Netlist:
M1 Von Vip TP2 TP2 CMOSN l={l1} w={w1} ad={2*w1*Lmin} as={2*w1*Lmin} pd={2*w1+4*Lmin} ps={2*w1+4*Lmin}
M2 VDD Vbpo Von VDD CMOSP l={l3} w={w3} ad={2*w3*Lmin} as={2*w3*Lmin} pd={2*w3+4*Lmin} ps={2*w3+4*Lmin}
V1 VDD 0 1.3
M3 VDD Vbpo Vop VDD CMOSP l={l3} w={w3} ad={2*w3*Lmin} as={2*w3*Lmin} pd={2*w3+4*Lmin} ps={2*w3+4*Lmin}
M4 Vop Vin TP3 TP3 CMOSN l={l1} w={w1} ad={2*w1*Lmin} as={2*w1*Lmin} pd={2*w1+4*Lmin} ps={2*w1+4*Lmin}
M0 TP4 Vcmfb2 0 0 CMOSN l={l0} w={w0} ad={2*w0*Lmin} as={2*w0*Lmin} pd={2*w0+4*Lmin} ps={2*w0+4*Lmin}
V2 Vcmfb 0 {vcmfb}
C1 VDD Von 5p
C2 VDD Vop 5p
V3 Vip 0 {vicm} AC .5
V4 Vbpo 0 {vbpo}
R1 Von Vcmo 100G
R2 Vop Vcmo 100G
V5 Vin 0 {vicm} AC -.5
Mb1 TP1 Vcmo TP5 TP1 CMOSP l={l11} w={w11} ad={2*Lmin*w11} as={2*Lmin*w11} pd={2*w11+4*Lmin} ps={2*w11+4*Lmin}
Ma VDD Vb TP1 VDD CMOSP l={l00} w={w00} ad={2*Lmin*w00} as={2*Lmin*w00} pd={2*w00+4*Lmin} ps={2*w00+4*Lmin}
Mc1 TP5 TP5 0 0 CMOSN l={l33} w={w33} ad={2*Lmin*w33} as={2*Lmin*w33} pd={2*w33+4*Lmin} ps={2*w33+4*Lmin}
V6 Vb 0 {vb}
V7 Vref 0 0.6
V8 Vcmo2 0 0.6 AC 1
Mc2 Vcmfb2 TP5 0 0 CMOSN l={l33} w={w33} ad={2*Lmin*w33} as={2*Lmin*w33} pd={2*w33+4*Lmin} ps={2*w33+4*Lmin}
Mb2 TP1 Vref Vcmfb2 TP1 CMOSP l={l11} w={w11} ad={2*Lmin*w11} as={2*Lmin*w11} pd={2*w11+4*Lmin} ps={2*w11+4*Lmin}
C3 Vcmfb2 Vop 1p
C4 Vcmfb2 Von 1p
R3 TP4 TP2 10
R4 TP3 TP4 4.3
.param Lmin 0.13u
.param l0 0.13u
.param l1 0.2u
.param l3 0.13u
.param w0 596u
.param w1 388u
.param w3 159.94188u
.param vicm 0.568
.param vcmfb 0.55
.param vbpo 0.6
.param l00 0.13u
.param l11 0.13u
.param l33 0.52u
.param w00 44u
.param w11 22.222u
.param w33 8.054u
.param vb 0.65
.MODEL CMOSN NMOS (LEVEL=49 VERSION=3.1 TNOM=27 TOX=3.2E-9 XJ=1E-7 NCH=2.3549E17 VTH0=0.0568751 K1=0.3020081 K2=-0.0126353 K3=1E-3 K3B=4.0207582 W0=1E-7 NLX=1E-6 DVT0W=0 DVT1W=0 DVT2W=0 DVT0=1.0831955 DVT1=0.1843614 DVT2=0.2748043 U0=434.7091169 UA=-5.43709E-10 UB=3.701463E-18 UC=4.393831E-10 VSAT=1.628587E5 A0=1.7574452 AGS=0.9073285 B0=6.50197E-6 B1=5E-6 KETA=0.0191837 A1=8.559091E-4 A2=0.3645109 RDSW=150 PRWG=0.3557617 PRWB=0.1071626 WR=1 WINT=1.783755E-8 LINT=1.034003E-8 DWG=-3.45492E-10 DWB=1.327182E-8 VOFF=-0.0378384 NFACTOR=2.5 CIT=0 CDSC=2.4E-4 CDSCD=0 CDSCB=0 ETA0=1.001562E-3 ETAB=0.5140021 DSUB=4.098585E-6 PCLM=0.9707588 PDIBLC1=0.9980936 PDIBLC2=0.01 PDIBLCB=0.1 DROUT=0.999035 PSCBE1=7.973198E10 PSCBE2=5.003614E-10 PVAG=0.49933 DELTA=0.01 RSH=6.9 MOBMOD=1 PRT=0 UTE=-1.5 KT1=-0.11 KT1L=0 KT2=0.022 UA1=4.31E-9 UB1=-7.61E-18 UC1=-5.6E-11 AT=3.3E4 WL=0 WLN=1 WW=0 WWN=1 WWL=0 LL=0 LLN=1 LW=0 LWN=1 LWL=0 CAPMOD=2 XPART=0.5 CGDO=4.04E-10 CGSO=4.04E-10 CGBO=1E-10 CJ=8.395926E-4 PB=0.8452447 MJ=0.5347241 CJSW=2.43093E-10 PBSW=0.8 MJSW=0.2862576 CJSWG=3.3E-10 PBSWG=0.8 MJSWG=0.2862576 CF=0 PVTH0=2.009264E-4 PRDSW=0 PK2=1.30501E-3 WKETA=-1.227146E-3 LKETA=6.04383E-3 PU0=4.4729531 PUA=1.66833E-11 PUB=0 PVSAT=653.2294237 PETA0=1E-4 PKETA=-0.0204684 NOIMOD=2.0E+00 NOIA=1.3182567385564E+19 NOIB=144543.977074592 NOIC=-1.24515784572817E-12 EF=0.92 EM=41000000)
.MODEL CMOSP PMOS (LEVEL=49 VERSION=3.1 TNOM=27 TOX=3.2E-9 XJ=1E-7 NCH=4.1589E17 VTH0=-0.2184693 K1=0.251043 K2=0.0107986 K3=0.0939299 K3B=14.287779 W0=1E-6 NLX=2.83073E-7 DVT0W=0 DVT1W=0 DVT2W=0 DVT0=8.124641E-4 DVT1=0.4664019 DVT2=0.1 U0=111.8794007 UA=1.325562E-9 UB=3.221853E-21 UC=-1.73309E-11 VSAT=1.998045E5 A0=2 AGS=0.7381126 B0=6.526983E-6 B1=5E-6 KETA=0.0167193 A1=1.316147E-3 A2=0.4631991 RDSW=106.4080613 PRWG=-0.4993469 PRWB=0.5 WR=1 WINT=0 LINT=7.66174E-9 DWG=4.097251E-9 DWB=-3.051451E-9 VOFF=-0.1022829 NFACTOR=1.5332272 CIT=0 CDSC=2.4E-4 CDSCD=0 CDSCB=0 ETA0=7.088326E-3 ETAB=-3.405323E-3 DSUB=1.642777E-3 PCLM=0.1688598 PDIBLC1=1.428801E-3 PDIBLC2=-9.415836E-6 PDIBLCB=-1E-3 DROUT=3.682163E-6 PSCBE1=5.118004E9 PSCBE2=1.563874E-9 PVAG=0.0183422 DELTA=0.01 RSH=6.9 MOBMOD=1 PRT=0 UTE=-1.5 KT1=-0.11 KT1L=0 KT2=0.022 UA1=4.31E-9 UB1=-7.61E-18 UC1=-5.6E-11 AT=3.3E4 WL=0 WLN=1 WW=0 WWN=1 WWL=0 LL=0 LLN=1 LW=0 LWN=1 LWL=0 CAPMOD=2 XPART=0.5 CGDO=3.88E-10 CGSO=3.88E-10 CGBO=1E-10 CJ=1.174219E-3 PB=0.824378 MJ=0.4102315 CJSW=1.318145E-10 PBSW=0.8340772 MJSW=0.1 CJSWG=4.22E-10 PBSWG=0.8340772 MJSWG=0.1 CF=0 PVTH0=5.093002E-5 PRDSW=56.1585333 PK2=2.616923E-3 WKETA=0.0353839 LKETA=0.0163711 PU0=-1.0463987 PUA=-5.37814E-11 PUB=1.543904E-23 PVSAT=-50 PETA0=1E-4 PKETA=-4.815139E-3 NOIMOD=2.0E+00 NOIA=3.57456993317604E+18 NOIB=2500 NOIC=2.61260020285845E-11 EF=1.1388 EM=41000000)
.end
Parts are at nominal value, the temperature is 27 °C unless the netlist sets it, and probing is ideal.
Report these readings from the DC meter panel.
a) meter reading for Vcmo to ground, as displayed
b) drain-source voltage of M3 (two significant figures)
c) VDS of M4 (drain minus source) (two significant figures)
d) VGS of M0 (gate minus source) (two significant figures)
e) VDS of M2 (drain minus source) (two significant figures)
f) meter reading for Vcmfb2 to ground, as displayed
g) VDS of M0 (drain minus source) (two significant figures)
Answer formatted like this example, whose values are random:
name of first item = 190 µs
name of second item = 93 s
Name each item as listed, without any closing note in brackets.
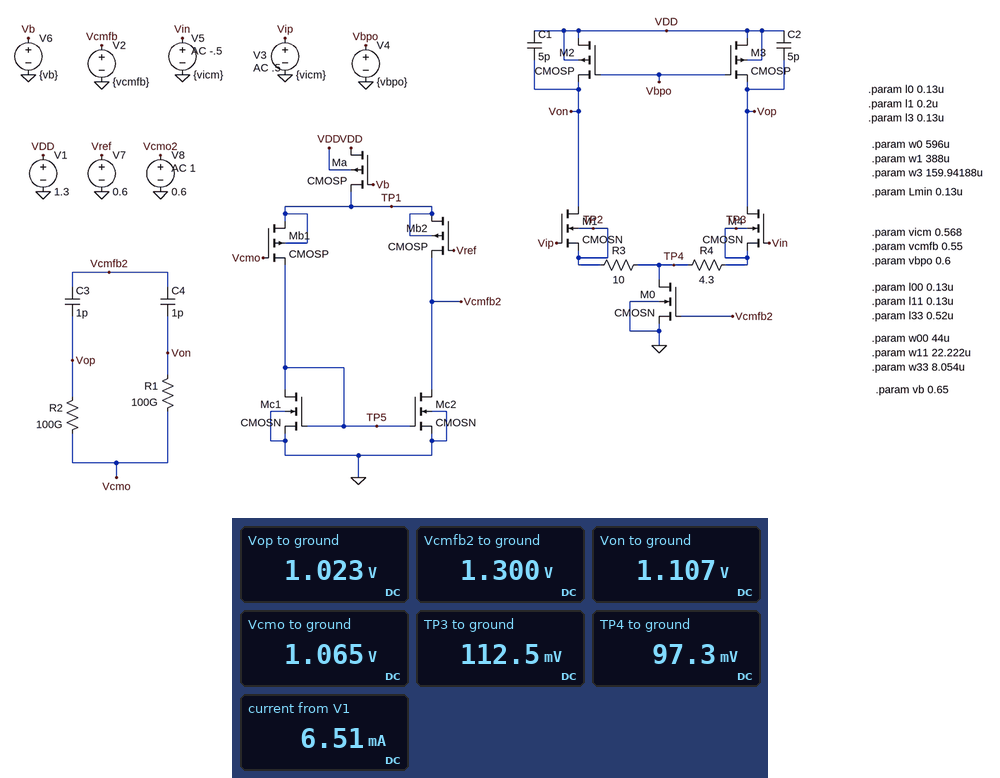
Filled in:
meter reading for Vcmo to ground, as displayed = 1.065 V
drain-source voltage of M3 = 280 mV
VDS of M4 (drain minus source) = 910 mV
VGS of M0 (gate minus source) = 1.3 V
VDS of M2 (drain minus source) = 190 mV
meter reading for Vcmfb2 to ground, as displayed = 1.300 V
VDS of M0 (drain minus source) = 97 mV
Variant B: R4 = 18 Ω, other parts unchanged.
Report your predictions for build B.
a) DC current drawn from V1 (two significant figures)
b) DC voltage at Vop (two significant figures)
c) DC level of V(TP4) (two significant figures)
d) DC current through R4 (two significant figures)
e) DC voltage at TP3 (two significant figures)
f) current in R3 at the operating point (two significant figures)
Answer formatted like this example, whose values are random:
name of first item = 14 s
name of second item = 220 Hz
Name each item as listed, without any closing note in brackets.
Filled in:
DC current drawn from V1 = 5.9 mA
DC voltage at Vop = 1.1 V
DC level of V(TP4) = 88 mV
DC current through R4 = 2.7 mA
DC voltage at TP3 = 140 mV
current in R3 at the operating point = 3.2 mA
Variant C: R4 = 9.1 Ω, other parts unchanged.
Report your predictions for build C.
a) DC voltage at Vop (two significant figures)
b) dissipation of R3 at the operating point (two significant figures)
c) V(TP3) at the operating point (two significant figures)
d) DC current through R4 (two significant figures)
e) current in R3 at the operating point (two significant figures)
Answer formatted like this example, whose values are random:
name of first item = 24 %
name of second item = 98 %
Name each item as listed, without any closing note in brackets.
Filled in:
DC voltage at Vop = 1.1 V
dissipation of R3 at the operating point = 95 µW
V(TP3) at the operating point = 120 mV
DC current through R4 = 3.2 mA
current in R3 at the operating point = 3.1 mA
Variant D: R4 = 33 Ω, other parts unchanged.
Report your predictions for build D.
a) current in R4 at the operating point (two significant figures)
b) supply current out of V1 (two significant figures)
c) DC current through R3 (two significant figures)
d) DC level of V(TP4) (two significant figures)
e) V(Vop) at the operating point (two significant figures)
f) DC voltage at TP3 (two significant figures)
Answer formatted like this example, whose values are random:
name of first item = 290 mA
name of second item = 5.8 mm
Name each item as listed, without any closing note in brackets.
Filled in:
current in R4 at the operating point = 2.1 mA
supply current out of V1 = 5.5 mA
DC current through R3 = 3.4 mA
DC level of V(TP4) = 82 mV
V(Vop) at the operating point = 1.2 V
DC voltage at TP3 = 150 mV
